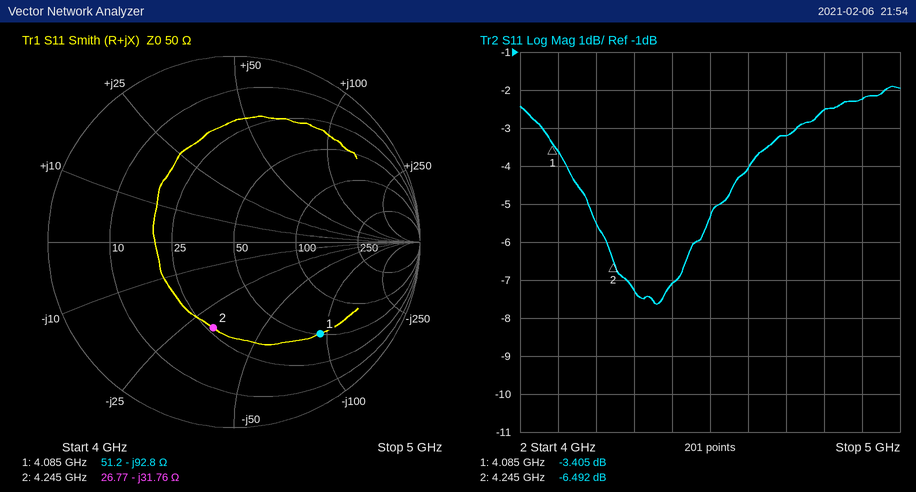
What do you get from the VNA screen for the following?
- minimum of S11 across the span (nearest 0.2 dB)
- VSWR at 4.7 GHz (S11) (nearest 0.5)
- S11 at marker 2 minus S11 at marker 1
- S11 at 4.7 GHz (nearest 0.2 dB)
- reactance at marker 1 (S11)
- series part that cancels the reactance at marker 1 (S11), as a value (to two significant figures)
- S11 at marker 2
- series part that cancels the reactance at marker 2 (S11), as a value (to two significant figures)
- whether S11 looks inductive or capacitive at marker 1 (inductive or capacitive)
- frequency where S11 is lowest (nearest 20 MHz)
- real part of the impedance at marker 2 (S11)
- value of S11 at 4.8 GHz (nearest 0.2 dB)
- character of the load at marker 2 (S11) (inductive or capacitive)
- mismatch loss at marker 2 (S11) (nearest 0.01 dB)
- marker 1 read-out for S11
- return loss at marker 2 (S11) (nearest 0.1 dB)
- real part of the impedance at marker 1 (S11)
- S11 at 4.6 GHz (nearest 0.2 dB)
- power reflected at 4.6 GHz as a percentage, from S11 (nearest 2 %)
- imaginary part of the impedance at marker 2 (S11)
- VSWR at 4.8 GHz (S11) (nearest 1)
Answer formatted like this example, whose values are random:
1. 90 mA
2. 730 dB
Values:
1. -7.6 dB
2. 5.5
3. -3.087 dB
4. -3.2 dB
5. -92.8 Ω
6. 3.6 nH
7. -6.492 dB
8. 1.2 nH
9. capacitive
10. 4.36 GHz
11. 26.77 Ω
12. -2.6 dB
13. capacitive
14. 1.10 dB
15. -3.405 dB
16. 6.5 dB
17. 51.2 Ω
18. -4.0 dB
19. 40 %
20. -31.76 Ω
21. 7
